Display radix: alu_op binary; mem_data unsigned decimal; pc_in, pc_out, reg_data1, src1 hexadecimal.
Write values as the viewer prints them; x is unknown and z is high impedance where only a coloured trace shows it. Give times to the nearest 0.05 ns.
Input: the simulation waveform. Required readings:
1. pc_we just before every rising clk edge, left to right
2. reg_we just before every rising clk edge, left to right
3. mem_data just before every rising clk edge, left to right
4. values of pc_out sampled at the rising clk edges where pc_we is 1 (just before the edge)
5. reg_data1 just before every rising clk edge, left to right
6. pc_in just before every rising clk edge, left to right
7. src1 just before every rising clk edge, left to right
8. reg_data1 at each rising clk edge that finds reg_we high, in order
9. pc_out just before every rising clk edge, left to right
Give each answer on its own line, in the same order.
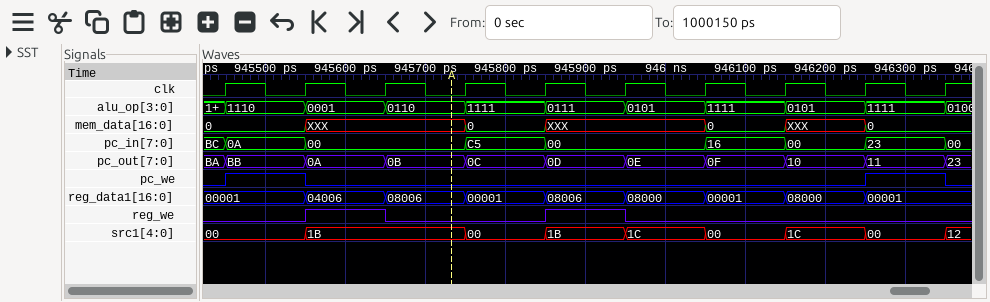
0 1 0 0 0 0 0 0 0 1
0 0 1 0 0 1 0 0 0 0
0, 0, XXX, XXX, 0, XXX, XXX, 0, XXX, 0
BB, 11
00001, 00001, 04006, 08006, 00001, 08006, 08000, 00001, 08000, 00001
BC, 0A, 00, 00, C5, 00, 00, 16, 00, 23
00, 00, 1B, 1B, 00, 1B, 1C, 00, 1C, 00
04006, 08006
BA, BB, 0A, 0B, 0C, 0D, 0E, 0F, 10, 11
